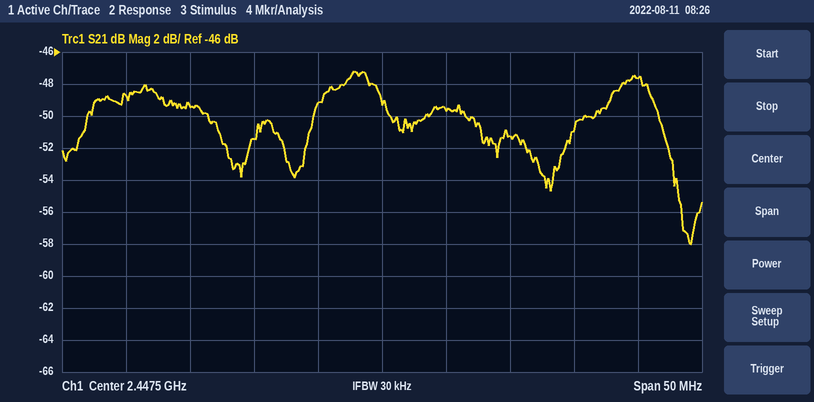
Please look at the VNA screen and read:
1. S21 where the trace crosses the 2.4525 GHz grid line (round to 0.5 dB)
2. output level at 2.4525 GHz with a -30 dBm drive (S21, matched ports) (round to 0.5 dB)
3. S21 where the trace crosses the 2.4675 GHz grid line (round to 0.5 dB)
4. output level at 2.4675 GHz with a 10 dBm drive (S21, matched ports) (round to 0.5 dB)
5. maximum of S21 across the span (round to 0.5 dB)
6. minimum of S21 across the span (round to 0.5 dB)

-49.5 dB
-79.5 dBm
-47.5 dB
-37.5 dBm
-47.0 dB
-58.0 dB
